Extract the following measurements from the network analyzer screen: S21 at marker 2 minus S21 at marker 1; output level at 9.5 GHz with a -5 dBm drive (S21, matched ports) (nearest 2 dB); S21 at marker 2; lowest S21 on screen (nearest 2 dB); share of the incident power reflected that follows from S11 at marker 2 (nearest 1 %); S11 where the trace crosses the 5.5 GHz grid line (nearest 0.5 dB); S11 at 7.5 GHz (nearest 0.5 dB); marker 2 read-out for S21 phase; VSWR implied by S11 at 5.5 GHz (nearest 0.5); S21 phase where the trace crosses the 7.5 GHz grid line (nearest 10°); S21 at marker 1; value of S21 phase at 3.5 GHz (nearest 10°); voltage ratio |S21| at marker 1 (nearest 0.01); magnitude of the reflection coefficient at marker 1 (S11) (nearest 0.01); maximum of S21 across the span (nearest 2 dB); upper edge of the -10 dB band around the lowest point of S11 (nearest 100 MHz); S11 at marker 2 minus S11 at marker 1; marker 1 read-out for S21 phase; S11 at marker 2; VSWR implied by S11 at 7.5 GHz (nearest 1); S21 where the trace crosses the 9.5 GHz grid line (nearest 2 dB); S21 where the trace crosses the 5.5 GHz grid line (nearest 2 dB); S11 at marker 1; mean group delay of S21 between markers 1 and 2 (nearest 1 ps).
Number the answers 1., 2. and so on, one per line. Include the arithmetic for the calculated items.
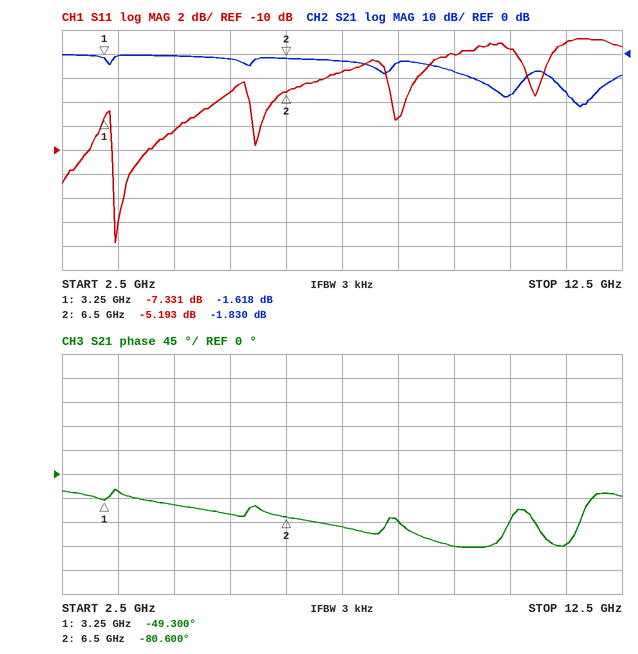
1. -1.83 − (-1.618) = -0.212 dB
2. -5 dBm + (-8 dB) = -12 dBm
3. -1.830 dB
4. -22 dB
5. 10^(-5.193/10) ≈ 30 %
6. -5.0 dB
7. -3.5 dB
8. -80.600°
9. |Γ| = 10^(-5/20) = 0.5623; VSWR = (1 + 0.5623)/(1 − 0.5623) ≈ 3.57, so 3.5 to the nearest 0.5
10. -100°
11. -1.618 dB
12. -30°
13. 10^(-1.618/20) ≈ 0.83
14. 10^(-7.331/20) ≈ 0.43
15. 0 dB
16. 4.0 GHz
17. -5.193 − (-7.331) = 2.138 dB
18. -49.300°
19. -5.193 dB
20. |Γ| = 10^(-3.5/20) = 0.6683; VSWR = (1 + 0.6683)/(1 − 0.6683) ≈ 5
21. -8 dB
22. -2 dB
23. -7.331 dB
24. −(-80.6° − (-49.3°))/(360° × 3.25 GHz) ≈ 27 ps
